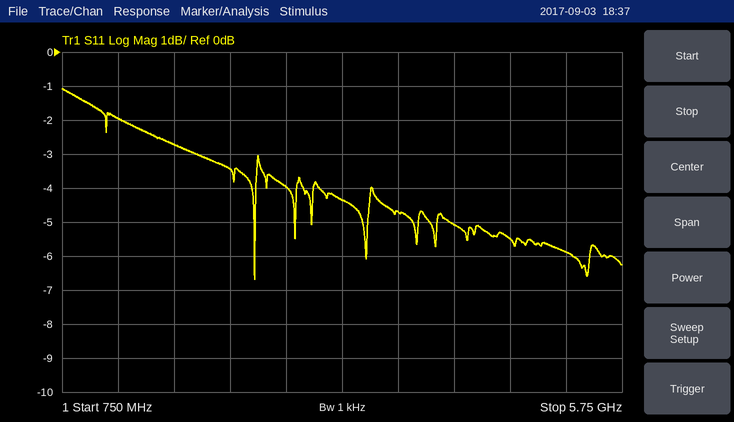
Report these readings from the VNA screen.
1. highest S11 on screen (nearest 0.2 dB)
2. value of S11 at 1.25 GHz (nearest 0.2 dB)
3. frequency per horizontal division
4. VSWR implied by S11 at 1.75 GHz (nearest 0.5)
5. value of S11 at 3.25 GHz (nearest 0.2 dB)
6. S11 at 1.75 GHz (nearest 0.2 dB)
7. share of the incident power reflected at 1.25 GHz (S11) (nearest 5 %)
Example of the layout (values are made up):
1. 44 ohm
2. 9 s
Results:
1. -1.0 dB
2. -2.0 dB
3. 500 MHz
4. 6.5
5. -4.4 dB
6. -2.8 dB
7. 65 %
